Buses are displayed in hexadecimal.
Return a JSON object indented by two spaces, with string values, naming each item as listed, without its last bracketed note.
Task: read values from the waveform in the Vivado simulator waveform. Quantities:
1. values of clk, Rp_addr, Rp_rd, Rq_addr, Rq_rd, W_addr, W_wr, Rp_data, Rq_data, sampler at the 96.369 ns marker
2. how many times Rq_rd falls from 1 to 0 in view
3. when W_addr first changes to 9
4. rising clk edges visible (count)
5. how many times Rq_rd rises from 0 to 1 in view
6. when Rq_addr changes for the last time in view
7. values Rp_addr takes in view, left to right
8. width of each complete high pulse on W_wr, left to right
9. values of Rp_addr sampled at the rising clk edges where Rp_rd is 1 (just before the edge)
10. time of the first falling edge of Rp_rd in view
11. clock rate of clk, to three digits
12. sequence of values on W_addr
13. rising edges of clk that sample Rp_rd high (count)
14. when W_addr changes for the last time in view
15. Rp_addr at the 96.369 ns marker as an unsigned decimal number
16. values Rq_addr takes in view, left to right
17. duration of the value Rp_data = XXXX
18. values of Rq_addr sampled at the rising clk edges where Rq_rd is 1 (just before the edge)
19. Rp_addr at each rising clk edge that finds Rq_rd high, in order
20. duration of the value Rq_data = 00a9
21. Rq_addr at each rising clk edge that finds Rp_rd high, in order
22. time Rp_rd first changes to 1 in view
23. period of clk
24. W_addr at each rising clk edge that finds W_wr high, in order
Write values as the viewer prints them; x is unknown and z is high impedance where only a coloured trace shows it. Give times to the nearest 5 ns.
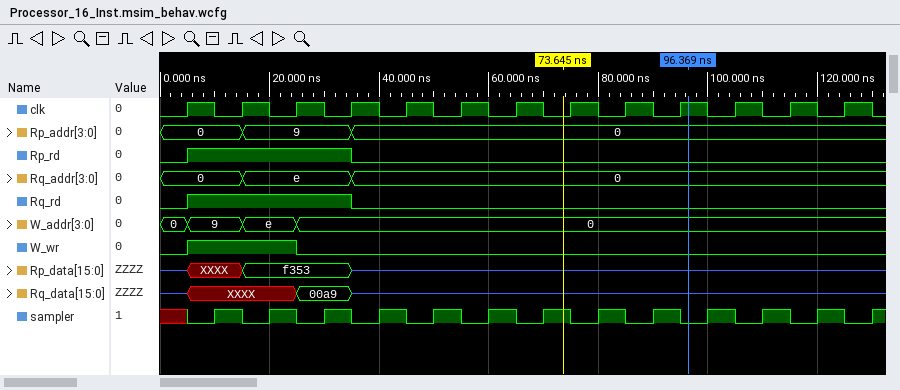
{
  "values of clk, Rp_addr, Rp_rd, Rq_addr, Rq_rd, W_addr, W_wr, Rp_data, Rq_data, sampler at the 96.369 ns marker": "clk=1, Rp_addr=0, Rp_rd=0, Rq_addr=0, Rq_rd=0, W_addr=0, W_wr=0, Rp_data=z, Rq_data=z, sampler=0",
  "how many times Rq_rd falls from 1 to 0 in view": "1",
  "when W_addr first changes to 9": "5 ns",
  "rising clk edges visible": "13",
  "how many times Rq_rd rises from 0 to 1 in view": "1",
  "when Rq_addr changes for the last time in view": "35 ns",
  "values Rp_addr takes in view, left to right": "0, 9, 0",
  "width of each complete high pulse on W_wr, left to right": "20 ns",
  "values of Rp_addr sampled at the rising clk edges where Rp_rd is 1": "0, 9, 9",
  "time of the first falling edge of Rp_rd in view": "35 ns",
  "clock rate of clk, to three digits": "100 MHz",
  "sequence of values on W_addr": "0, 9, e, 0",
  "rising edges of clk that sample Rp_rd high": "3",
  "when W_addr changes for the last time in view": "25 ns",
  "Rp_addr at the 96.369 ns marker as an unsigned decimal number": "0",
  "values Rq_addr takes in view, left to right": "0, e, 0",
  "duration of the value Rp_data = XXXX": "10 ns",
  "values of Rq_addr sampled at the rising clk edges where Rq_rd is 1": "0, e, e",
  "Rp_addr at each rising clk edge that finds Rq_rd high, in order": "0, 9, 9",
  "duration of the value Rq_data = 00a9": "10 ns",
  "Rq_addr at each rising clk edge that finds Rp_rd high, in order": "0, e, e",
  "time Rp_rd first changes to 1 in view": "5 ns",
  "period of clk": "10 ns",
  "W_addr at each rising clk edge that finds W_wr high, in order": "9, e"
}
